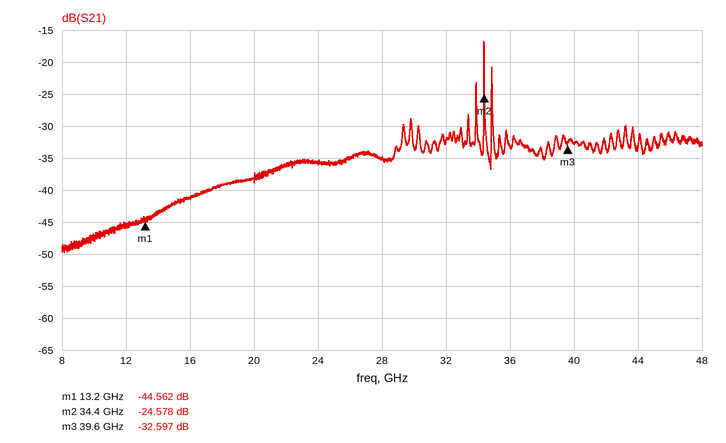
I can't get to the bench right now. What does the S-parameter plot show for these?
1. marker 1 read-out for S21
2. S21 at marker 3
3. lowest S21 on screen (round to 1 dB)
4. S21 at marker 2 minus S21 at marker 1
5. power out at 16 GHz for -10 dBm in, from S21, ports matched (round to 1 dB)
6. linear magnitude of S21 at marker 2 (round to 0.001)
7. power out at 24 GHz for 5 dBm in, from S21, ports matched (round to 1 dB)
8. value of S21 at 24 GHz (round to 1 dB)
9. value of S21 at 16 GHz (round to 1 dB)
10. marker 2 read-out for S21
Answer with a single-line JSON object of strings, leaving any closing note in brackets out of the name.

{"marker 1 read-out for S21": "-44.562 dB", "S21 at marker 3": "-32.597 dB", "lowest S21 on screen": "-50 dB", "S21 at marker 2 minus S21 at marker 1": "19.984 dB", "power out at 16 GHz for -10 dBm in, from S21, ports matched": "-51 dBm", "linear magnitude of S21 at marker 2": "0.059", "power out at 24 GHz for 5 dBm in, from S21, ports matched": "-31 dBm", "value of S21 at 24 GHz": "-36 dB", "value of S21 at 16 GHz": "-41 dB", "marker 2 read-out for S21": "-24.578 dB"}
